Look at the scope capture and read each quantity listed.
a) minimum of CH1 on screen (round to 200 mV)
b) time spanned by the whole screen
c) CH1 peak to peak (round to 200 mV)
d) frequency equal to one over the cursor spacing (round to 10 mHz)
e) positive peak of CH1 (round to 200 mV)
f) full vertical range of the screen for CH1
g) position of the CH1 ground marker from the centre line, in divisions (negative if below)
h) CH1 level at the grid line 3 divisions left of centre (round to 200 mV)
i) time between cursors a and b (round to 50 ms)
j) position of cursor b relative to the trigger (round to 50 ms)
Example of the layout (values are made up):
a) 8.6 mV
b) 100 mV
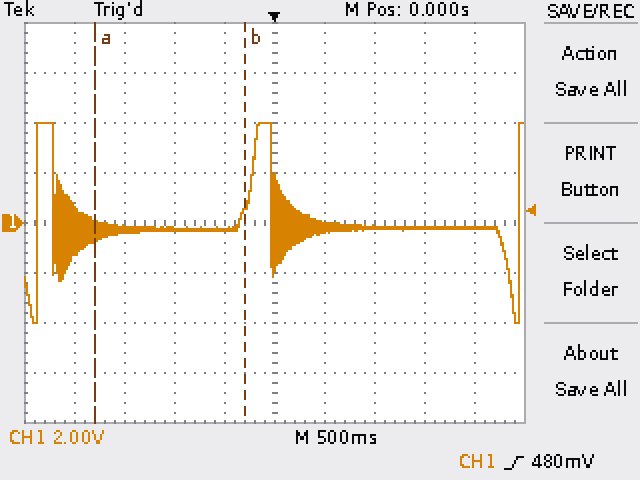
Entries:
a) -4.0 V
b) 5 s
c) 8.0 V
d) 670 mHz
e) 4.0 V
f) 16 V
g) 0.0 div
h) -200 mV
i) 1.50 s
j) -300 ms
